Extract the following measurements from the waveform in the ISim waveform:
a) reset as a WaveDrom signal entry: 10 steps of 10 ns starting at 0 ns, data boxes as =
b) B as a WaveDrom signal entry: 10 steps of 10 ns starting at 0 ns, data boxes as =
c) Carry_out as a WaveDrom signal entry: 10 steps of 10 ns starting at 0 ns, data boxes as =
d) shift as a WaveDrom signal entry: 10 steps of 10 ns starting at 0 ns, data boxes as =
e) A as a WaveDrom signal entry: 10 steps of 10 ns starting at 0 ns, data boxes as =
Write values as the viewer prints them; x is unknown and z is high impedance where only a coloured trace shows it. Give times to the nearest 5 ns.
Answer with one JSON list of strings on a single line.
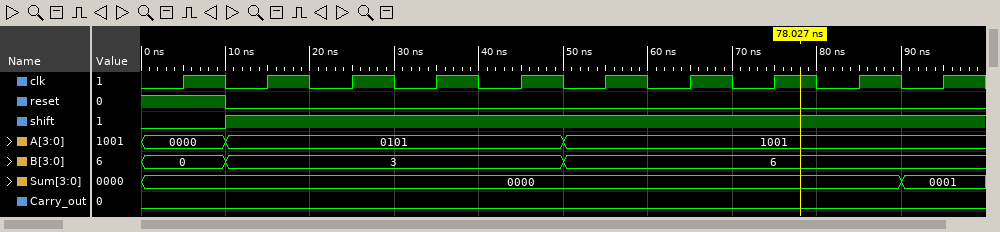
["{name: 'reset', wave: '10........'}", "{name: 'B', wave: '==...=....', data: '0 3 6'}", "{name: 'Carry_out', wave: '0.........'}", "{name: 'shift', wave: '01........'}", "{name: 'A', wave: '==...=....', data: '0000 0101 1001'}"]
